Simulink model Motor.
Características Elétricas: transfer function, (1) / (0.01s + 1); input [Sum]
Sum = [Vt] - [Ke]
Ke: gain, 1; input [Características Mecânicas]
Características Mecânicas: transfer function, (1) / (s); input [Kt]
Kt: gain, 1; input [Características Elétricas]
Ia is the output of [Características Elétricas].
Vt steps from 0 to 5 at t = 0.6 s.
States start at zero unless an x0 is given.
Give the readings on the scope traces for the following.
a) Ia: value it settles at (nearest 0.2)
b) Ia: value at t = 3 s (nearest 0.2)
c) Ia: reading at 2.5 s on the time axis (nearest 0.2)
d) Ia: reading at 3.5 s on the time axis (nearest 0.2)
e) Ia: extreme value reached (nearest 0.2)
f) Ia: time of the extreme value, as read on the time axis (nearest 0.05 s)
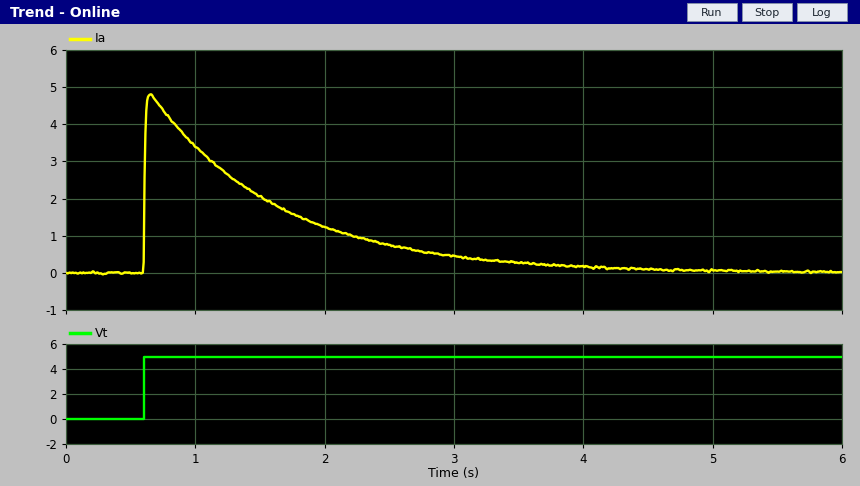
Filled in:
0.0
0.4
0.8
0.2
4.8
0.65 s
